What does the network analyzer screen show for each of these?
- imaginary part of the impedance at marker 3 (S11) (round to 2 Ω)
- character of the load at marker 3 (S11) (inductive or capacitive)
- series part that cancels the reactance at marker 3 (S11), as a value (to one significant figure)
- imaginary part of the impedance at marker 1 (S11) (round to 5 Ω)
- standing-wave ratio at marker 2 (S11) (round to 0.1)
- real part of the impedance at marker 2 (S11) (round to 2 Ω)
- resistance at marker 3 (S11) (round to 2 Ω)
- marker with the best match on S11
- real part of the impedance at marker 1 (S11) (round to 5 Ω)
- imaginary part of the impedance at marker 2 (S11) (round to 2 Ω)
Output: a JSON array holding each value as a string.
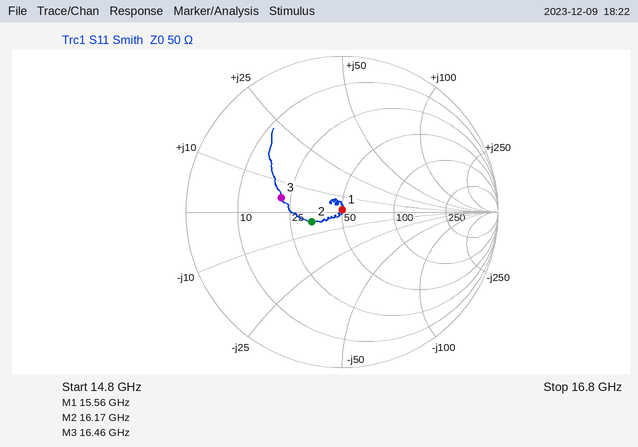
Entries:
["+4 Ω", "inductive", "2 pF", "0 Ω", "1.5", "34 Ω", "22 Ω", "marker 1", "50 Ω", "-4 Ω"]
